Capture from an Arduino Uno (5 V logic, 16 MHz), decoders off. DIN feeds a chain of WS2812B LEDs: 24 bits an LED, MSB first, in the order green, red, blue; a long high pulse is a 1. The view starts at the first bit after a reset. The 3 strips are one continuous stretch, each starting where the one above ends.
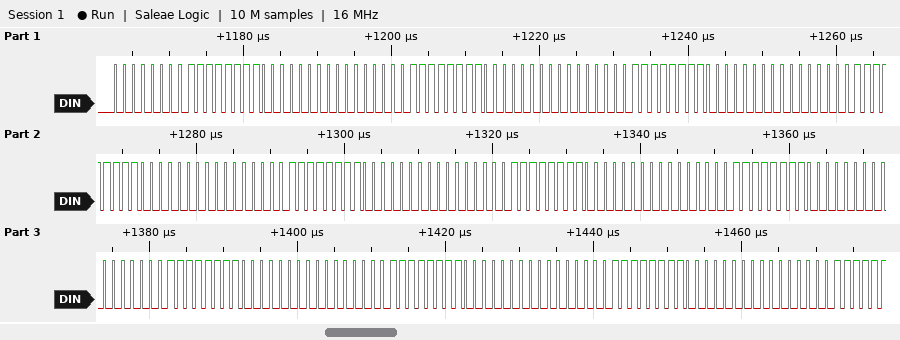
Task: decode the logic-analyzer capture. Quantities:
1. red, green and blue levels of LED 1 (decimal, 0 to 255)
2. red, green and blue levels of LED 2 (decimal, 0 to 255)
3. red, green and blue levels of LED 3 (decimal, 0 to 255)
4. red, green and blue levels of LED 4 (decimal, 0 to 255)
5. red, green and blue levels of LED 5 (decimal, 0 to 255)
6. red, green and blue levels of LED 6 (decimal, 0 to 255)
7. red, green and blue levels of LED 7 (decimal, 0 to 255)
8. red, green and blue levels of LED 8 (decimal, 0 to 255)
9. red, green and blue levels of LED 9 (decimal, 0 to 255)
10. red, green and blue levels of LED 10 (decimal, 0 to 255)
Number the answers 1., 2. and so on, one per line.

1. 255, 0, 0
2. 255, 0, 0
3. 255, 0, 0
4. 255, 0, 0
5. 255, 0, 0
6. 255, 0, 0
7. 255, 0, 0
8. 255, 0, 0
9. 255, 0, 0
10. 255, 0, 0
